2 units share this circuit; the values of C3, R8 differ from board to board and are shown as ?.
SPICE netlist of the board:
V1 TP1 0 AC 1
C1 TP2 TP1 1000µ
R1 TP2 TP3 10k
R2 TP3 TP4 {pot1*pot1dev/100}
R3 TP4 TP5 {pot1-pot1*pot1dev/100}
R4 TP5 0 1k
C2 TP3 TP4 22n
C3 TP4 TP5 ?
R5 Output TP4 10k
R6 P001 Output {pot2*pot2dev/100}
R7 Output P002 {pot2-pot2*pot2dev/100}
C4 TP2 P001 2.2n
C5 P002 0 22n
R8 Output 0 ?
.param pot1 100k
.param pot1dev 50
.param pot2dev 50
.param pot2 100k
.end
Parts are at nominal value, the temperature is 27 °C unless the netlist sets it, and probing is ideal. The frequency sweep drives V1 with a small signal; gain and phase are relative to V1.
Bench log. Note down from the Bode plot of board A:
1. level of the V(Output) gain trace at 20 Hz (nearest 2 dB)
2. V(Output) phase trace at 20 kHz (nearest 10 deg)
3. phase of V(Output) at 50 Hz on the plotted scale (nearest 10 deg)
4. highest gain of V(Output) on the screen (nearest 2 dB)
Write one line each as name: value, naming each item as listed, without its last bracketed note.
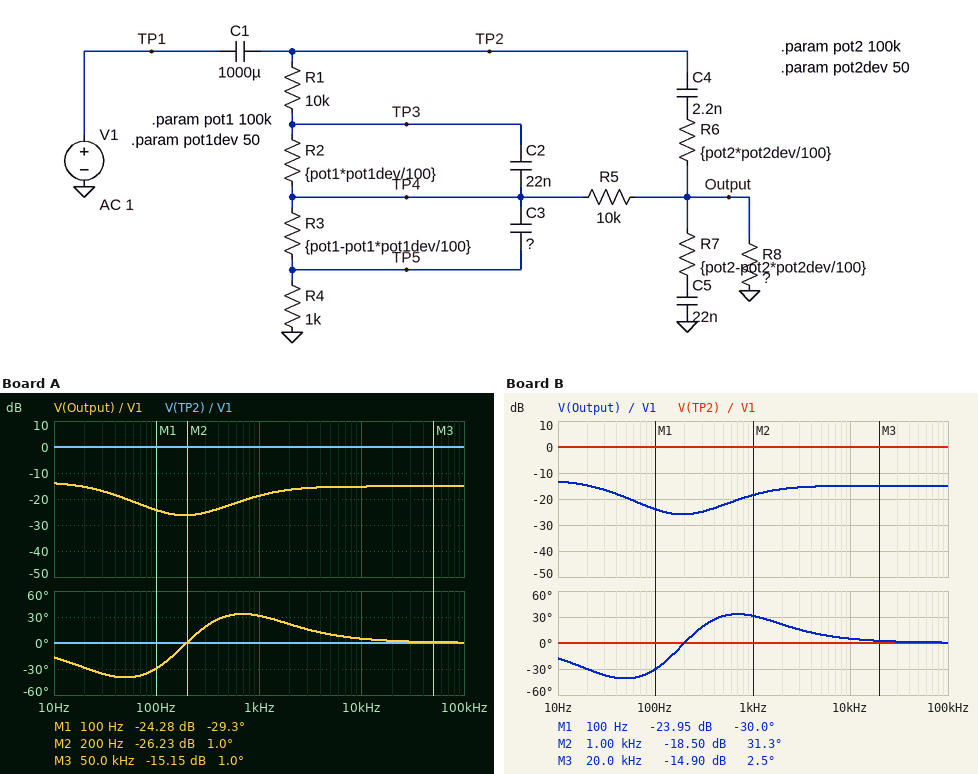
level of the V(Output) gain trace at 20 Hz: -16 dB
V(Output) phase trace at 20 kHz: 0 deg
phase of V(Output) at 50 Hz on the plotted scale: -40 deg
highest gain of V(Output) on the screen: -14 dB
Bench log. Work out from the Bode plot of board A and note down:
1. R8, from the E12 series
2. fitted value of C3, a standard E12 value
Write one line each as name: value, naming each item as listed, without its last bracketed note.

R8, from the E12 series: 33 kΩ
fitted value of C3, a standard E12 value: 330 nF
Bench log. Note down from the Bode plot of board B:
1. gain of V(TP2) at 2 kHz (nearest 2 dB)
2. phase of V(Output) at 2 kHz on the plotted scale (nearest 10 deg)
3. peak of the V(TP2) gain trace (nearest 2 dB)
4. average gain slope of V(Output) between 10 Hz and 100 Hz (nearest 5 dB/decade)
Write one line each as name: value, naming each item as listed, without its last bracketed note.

gain of V(TP2) at 2 kHz: 0 dB
phase of V(Output) at 2 kHz on the plotted scale: 20 deg
peak of the V(TP2) gain trace: 0 dB
average gain slope of V(Output) between 10 Hz and 100 Hz: -10 dB/decade
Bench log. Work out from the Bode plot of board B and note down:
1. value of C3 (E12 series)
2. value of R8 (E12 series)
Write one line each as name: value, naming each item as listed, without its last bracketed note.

value of C3: 330 nF
value of R8: 39 kΩ
